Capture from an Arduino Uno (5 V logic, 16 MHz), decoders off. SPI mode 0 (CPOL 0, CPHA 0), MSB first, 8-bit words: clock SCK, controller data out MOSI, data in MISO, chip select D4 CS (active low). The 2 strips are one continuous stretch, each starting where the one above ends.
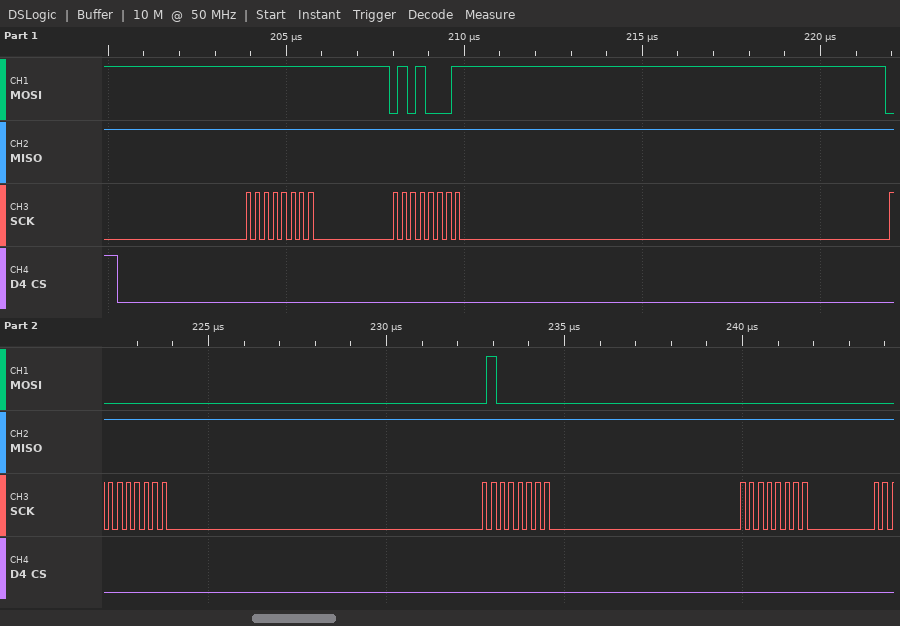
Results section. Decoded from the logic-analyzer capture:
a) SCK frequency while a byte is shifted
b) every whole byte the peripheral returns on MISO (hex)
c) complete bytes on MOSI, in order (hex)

4 MHz
0xFF 0xFF 0xFF 0xFF 0xFF
0xFF 0x51 0x00 0x40 0x00
